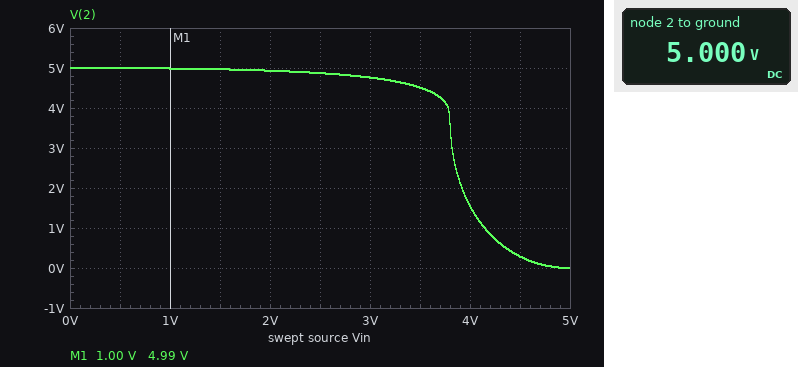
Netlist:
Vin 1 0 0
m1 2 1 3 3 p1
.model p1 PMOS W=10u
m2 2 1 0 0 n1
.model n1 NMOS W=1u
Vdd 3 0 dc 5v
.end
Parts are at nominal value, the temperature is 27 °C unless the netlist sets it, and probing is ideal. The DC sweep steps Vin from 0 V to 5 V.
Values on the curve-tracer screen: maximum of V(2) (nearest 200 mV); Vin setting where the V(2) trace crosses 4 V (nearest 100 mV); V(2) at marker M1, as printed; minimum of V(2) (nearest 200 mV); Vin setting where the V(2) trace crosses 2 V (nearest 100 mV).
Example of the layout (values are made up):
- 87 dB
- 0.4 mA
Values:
- 5.0 V
- 3.8 V
- 4.99 V
- 0 V
- 3.9 V
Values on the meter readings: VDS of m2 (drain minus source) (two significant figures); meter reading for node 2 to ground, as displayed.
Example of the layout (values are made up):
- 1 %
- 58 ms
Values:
- 5.0 V
- 5.000 V
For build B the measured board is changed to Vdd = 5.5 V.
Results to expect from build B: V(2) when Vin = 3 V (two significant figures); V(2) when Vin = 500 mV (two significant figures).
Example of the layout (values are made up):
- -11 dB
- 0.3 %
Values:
- 5.3 V
- 5.5 V
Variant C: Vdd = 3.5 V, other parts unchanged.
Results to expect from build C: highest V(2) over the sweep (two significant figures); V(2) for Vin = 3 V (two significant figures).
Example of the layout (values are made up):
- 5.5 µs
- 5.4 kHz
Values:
- 3.5 V
- 450 mV
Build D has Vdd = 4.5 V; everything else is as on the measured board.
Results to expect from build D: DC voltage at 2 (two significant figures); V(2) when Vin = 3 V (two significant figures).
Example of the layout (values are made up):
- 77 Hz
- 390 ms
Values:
- 4.5 V
- 4.2 V
